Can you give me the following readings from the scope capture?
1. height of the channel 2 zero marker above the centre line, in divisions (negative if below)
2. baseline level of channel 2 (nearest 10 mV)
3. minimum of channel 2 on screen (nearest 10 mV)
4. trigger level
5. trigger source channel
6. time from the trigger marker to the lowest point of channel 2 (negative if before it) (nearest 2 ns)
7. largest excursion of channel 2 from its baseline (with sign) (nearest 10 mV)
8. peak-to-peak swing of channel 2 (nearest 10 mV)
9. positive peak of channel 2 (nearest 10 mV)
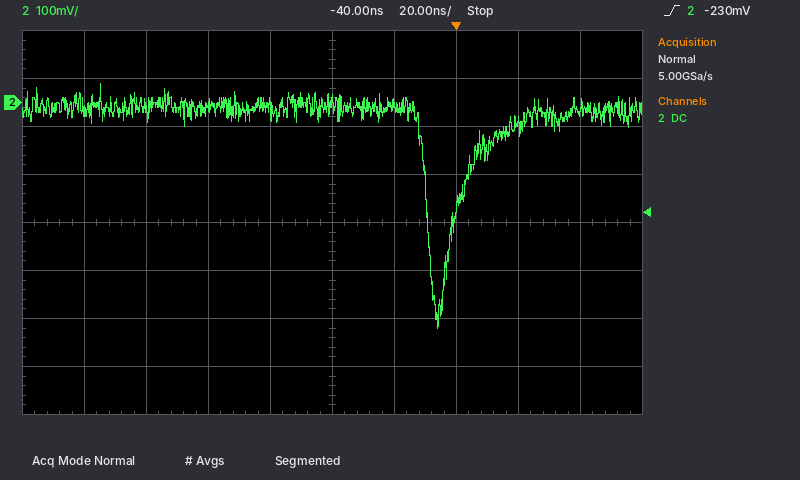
+2.5 div
-10 mV
-470 mV
-230 mV
channel 2
-6 ns
-460 mV
510 mV
40 mV
